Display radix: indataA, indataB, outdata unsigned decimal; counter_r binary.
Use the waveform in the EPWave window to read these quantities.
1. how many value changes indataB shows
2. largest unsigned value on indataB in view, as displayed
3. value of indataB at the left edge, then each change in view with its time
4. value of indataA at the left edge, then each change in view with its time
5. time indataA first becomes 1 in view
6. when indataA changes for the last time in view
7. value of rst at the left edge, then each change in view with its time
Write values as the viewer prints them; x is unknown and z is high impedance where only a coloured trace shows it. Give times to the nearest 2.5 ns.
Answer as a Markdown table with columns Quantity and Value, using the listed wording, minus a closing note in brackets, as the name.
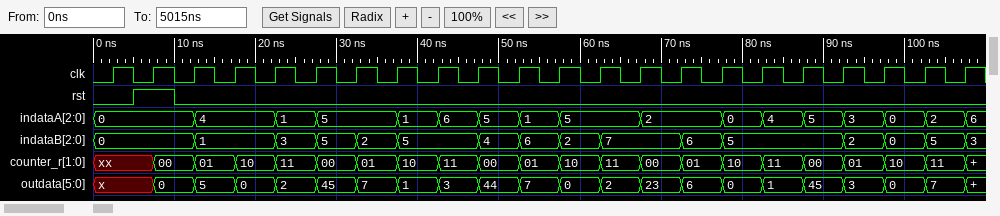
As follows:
| Quantity | Value |
|---|---|
| how many value changes indataB shows | 15 |
| largest unsigned value on indataB in view, as displayed | 7 |
| value of indataB at the left edge, then each change in view with its time | 0, 1 at 12.5 ns, 3 at 22.5 ns, 5 at 27.5 ns, 2 at 32.5 ns, 5 at 37.5 ns, 4 at 47.5 ns, 6 at 52.5 ns, 2 at 57.5 ns, 7 at 62.5 ns, 6 at 72.5 ns, 5 at 77.5 ns, 2 at 92.5 ns, 0 at 97.5 ns, 5 at 102.5 ns, 3 at 107.5 ns |
| value of indataA at the left edge, then each change in view with its time | 0, 4 at 12.5 ns, 1 at 22.5 ns, 5 at 27.5 ns, 1 at 37.5 ns, 6 at 42.5 ns, 5 at 47.5 ns, 1 at 52.5 ns, 5 at 57.5 ns, 2 at 67.5 ns, 0 at 77.5 ns, 4 at 82.5 ns, 5 at 87.5 ns, 3 at 92.5 ns, 0 at 97.5 ns, 2 at 102.5 ns, 6 at 107.5 ns |
| time indataA first becomes 1 in view | 22.5 ns |
| when indataA changes for the last time in view | 107.5 ns |
| value of rst at the left edge, then each change in view with its time | 0, 1 at 5 ns, 0 at 10 ns |
